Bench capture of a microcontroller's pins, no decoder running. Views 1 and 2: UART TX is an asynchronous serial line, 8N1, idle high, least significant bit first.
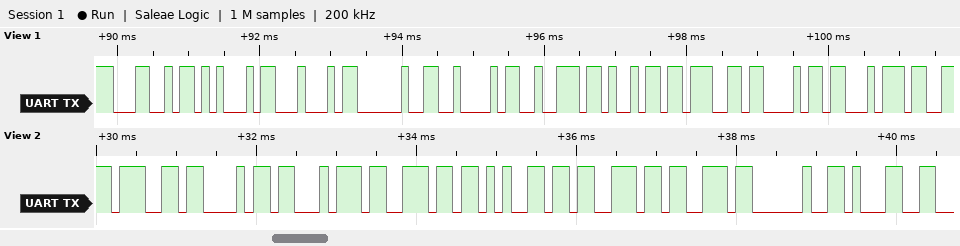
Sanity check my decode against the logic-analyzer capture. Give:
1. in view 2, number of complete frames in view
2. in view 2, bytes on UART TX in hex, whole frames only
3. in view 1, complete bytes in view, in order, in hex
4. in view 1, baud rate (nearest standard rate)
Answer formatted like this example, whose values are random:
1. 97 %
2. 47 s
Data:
1. 9
2. 67 68 74 6E 65 73 73 20 31
3. 4C 45 44 20 42 72 69 67 68 74
4. 9600 baud
